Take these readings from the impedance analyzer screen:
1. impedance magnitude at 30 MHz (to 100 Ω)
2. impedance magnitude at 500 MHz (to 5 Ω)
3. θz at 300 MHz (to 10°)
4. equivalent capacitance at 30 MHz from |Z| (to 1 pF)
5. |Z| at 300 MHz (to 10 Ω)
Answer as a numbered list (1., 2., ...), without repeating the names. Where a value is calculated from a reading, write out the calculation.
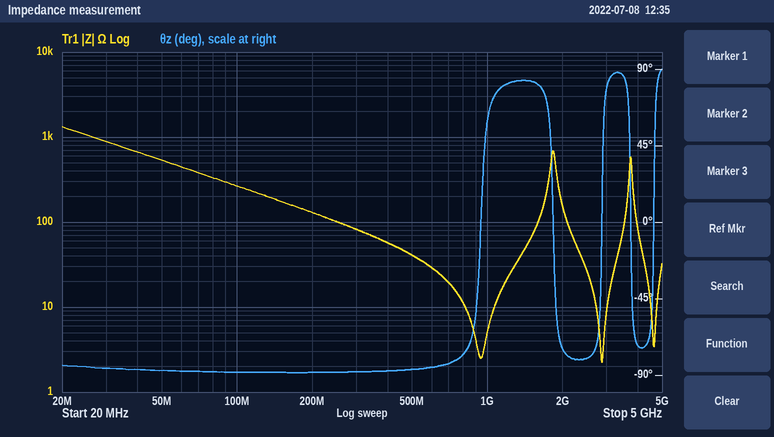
1. 900 Ω
2. 40 Ω
3. -90°
4. C = 1/(2π × 30 MHz × 900 Ω) ≈ 6 pF
5. 80 Ω
